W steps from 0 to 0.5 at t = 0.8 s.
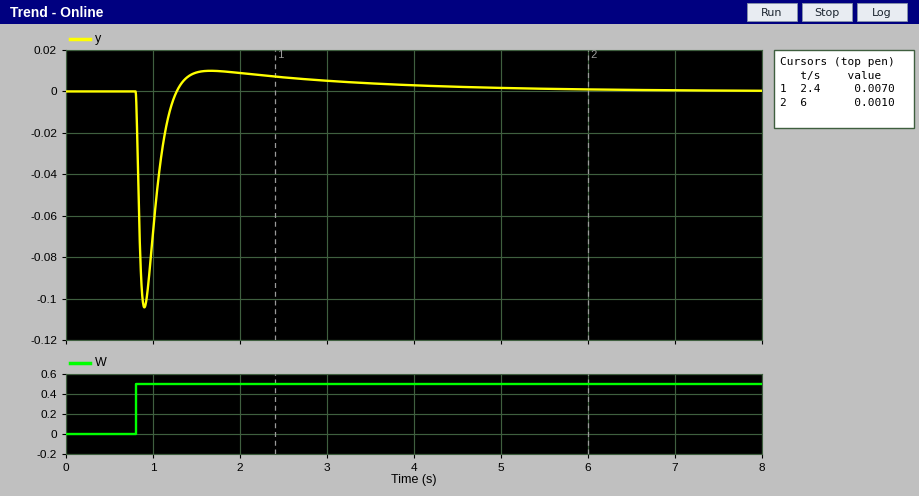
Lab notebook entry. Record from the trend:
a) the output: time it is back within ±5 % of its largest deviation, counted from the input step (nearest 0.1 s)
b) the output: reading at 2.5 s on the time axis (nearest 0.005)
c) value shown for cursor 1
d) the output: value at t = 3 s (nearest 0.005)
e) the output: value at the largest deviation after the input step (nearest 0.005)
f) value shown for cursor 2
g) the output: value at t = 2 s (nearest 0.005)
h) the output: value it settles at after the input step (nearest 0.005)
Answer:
2.2 s
0.005
0.0070
0.005
-0.105
0.0010
0.010
0.000
